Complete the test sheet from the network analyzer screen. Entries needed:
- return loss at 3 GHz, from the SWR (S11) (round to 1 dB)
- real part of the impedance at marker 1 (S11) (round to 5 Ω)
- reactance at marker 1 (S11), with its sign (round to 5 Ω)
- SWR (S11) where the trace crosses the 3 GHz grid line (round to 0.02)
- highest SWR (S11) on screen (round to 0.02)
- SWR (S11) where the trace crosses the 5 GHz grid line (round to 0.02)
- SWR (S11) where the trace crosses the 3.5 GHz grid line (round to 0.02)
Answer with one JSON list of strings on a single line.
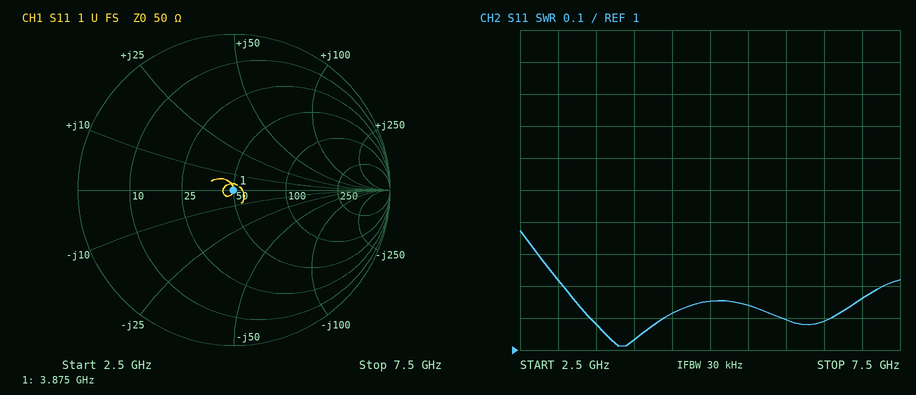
["20 dB", "50 Ω", "0 Ω", "1.22", "1.38", "1.16", "1.08"]
